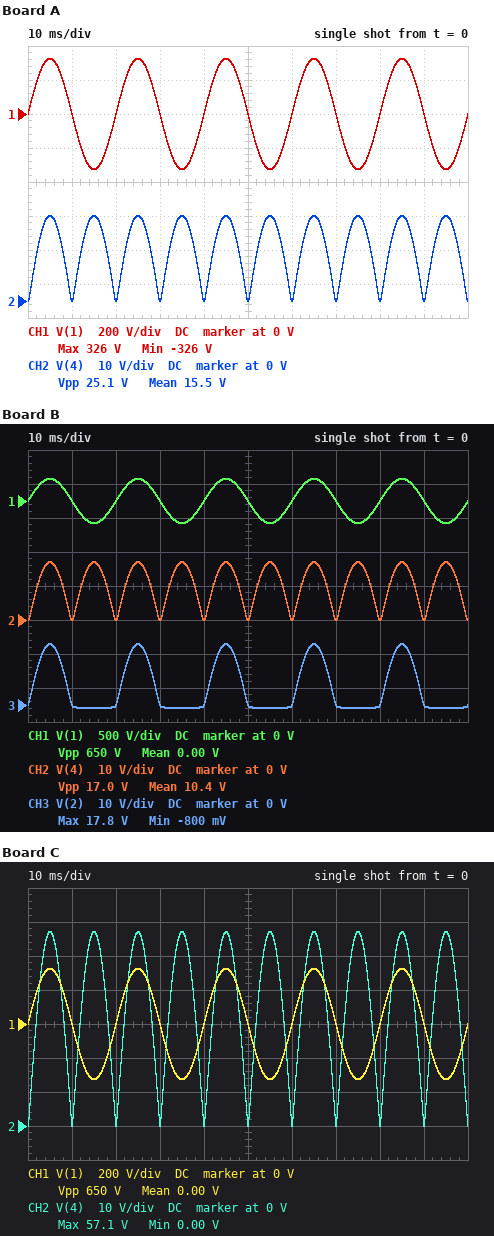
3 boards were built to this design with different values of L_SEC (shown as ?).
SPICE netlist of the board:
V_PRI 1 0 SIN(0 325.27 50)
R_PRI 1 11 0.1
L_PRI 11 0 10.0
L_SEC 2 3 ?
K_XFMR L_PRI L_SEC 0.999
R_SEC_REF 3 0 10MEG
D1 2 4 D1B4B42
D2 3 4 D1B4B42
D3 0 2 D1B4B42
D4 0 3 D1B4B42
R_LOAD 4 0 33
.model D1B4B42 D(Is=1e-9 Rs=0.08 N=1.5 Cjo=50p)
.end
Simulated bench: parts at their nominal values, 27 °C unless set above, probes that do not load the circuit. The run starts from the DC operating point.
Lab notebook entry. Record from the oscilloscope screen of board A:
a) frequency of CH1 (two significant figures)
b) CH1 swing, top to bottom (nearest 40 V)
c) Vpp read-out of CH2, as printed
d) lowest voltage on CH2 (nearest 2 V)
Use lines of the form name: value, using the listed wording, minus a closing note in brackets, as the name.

frequency of CH1: 50 Hz
CH1 swing, top to bottom: 640 V
Vpp read-out of CH2, as printed: 25.1 V
lowest voltage on CH2: 0 V
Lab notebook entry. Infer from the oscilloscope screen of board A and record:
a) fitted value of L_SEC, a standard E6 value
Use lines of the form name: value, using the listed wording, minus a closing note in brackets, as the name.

fitted value of L_SEC, a standard E6 value: 68 mH
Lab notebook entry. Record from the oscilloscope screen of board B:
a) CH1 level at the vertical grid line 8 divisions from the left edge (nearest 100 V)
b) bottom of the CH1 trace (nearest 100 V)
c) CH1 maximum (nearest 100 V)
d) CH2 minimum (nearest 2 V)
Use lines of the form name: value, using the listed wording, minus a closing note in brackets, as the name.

CH1 level at the vertical grid line 8 divisions from the left edge: 0 V
bottom of the CH1 trace: -300 V
CH1 maximum: 300 V
CH2 minimum: 0 V
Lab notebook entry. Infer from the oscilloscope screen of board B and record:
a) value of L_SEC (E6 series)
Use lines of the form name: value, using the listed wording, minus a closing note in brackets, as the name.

value of L_SEC: 33 mH
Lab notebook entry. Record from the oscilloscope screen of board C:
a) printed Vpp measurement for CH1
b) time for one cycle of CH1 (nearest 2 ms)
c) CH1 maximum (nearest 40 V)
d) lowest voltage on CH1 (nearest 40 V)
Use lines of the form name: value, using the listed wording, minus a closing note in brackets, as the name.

printed Vpp measurement for CH1: 650 V
time for one cycle of CH1: 20 ms
CH1 maximum: 320 V
lowest voltage on CH1: -320 V
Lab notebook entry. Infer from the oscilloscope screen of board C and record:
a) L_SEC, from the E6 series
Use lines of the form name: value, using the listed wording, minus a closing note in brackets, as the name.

L_SEC, from the E6 series: 330 mH
